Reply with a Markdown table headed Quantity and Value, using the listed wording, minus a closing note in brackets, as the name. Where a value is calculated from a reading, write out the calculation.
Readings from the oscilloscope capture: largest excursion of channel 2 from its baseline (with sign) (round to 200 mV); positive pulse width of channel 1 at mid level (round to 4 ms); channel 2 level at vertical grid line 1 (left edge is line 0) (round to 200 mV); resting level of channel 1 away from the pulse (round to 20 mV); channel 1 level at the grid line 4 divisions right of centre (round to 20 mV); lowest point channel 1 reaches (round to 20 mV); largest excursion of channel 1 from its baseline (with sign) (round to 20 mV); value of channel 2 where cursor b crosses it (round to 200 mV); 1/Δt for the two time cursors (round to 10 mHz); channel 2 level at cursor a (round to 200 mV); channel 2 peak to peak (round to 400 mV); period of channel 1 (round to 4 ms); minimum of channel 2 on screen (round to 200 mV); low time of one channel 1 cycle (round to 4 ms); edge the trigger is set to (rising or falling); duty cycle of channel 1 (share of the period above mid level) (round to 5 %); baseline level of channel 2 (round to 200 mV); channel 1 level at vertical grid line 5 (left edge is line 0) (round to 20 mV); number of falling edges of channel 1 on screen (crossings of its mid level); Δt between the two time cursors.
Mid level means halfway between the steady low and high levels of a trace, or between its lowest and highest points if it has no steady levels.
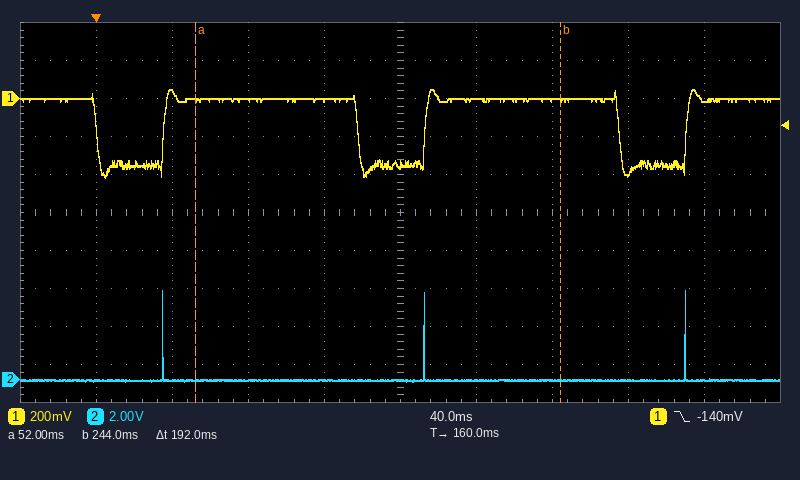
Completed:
| Quantity | Value |
|---|---|
| largest excursion of channel 2 from its baseline (with sign) | +4.8 V |
| positive pulse width of channel 1 at mid level | 104 ms |
| channel 2 level at vertical grid line 1 (left edge is line 0) | 0.0 V |
| resting level of channel 1 away from the pulse | 0 mV |
| channel 1 level at the grid line 4 divisions right of centre | 0 mV |
| lowest point channel 1 reaches | -420 mV |
| largest excursion of channel 1 from its baseline (with sign) | -420 mV − (0 mV) = -420 mV |
| value of channel 2 where cursor b crosses it | 0.0 V |
| 1/Δt for the two time cursors | 1 / 192 ms ≈ 5.21 Hz |
| channel 2 level at cursor a | 0.0 V |
| channel 2 peak to peak | 4.8 V |
| period of channel 1 | 136 ms |
| minimum of channel 2 on screen | 0.0 V |
| low time of one channel 1 cycle | 36 ms |
| edge the trigger is set to | falling |
| duty cycle of channel 1 (share of the period above mid level) | 104 ms / 136 ms ≈ 76.5 %, so 75 % to the nearest 5 % |
| baseline level of channel 2 | 0.0 V |
| channel 1 level at vertical grid line 5 (left edge is line 0) | -340 mV |
| number of falling edges of channel 1 on screen | 3 |
| Δt between the two time cursors | 192 ms |
